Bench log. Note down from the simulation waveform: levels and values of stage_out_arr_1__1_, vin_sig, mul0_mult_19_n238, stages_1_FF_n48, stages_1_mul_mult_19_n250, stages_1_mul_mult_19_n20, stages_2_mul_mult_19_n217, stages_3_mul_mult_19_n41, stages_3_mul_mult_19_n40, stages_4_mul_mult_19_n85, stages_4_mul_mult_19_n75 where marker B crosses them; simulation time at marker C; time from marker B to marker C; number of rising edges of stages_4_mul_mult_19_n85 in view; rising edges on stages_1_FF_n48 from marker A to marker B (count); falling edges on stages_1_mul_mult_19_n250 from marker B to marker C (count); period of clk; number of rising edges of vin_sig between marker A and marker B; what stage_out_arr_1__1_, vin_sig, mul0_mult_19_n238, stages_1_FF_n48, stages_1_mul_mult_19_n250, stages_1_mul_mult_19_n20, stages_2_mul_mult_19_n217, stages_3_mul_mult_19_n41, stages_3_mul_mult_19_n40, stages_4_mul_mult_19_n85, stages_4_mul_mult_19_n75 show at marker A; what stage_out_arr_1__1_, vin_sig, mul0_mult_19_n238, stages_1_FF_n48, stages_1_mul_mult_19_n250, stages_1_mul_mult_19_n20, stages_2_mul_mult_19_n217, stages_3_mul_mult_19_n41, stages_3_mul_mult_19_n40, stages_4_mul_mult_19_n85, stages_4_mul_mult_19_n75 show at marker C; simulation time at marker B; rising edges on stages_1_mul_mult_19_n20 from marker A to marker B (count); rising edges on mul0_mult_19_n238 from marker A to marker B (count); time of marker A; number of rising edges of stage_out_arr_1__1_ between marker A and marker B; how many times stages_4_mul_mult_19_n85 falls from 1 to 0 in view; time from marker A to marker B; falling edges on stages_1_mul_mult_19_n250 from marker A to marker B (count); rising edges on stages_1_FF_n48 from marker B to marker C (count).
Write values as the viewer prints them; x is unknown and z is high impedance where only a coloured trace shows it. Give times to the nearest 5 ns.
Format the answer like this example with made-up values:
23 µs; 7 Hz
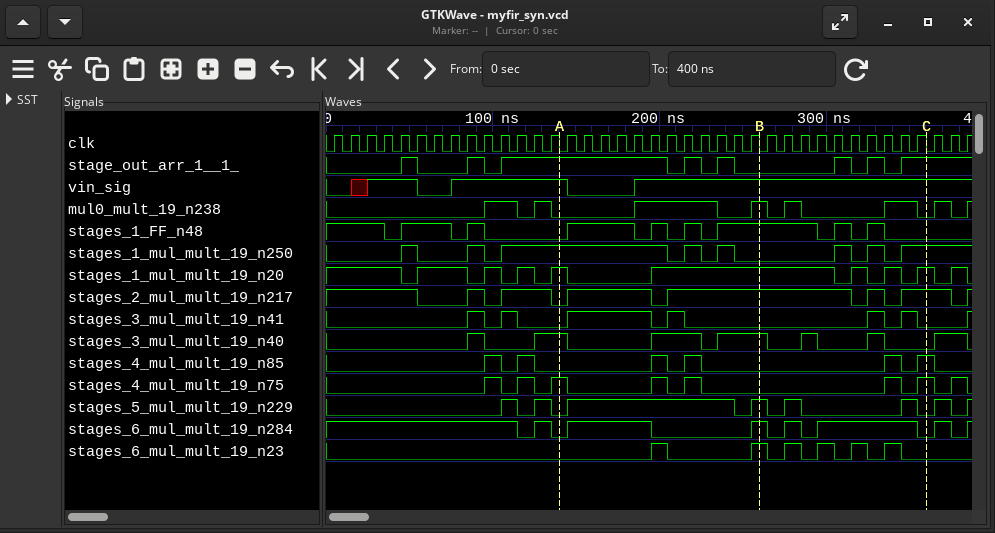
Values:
stage_out_arr_1__1_=0, vin_sig=1, mul0_mult_19_n238=1, stages_1_FF_n48=1, stages_1_mul_mult_19_n250=0, stages_1_mul_mult_19_n20=1, stages_2_mul_mult_19_n217=1, stages_3_mul_mult_19_n41=0, stages_3_mul_mult_19_n40=1, stages_4_mul_mult_19_n85=0, stages_4_mul_mult_19_n75=0; 360 ns; 100 ns; 6; 4; 2; 10 ns; 1; stage_out_arr_1__1_=1, vin_sig=1, mul0_mult_19_n238=0, stages_1_FF_n48=0, stages_1_mul_mult_19_n250=1, stages_1_mul_mult_19_n20=1, stages_2_mul_mult_19_n217=0, stages_3_mul_mult_19_n41=0, stages_3_mul_mult_19_n40=1, stages_4_mul_mult_19_n85=0, stages_4_mul_mult_19_n75=1; stage_out_arr_1__1_=1, vin_sig=1, mul0_mult_19_n238=0, stages_1_FF_n48=0, stages_1_mul_mult_19_n250=1, stages_1_mul_mult_19_n20=1, stages_2_mul_mult_19_n217=1, stages_3_mul_mult_19_n41=0, stages_3_mul_mult_19_n40=0, stages_4_mul_mult_19_n85=1, stages_4_mul_mult_19_n75=1; 260 ns; 1; 2; 140 ns; 2; 6; 120 ns; 3; 2
